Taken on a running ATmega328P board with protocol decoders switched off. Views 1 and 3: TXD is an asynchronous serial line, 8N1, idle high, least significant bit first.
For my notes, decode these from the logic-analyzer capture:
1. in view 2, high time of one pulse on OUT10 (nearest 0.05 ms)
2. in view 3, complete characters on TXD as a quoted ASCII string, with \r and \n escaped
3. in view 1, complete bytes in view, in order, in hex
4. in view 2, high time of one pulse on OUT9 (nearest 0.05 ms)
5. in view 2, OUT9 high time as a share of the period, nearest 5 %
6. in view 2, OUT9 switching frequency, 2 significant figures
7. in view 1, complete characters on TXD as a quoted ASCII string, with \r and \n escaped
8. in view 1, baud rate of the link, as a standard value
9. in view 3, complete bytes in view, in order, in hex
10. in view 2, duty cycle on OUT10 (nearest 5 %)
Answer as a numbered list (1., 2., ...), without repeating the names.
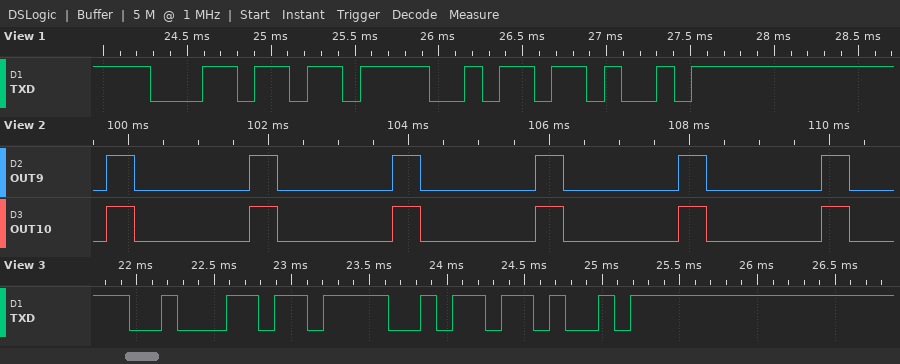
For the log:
1. 0.40 ms
2. "bOK"
3. 6C 4F 4B
4. 0.40 ms
5. 20 %
6. 490 Hz
7. "lOK"
8. 9600 baud
9. 62 4F 4B
10. 20 %
